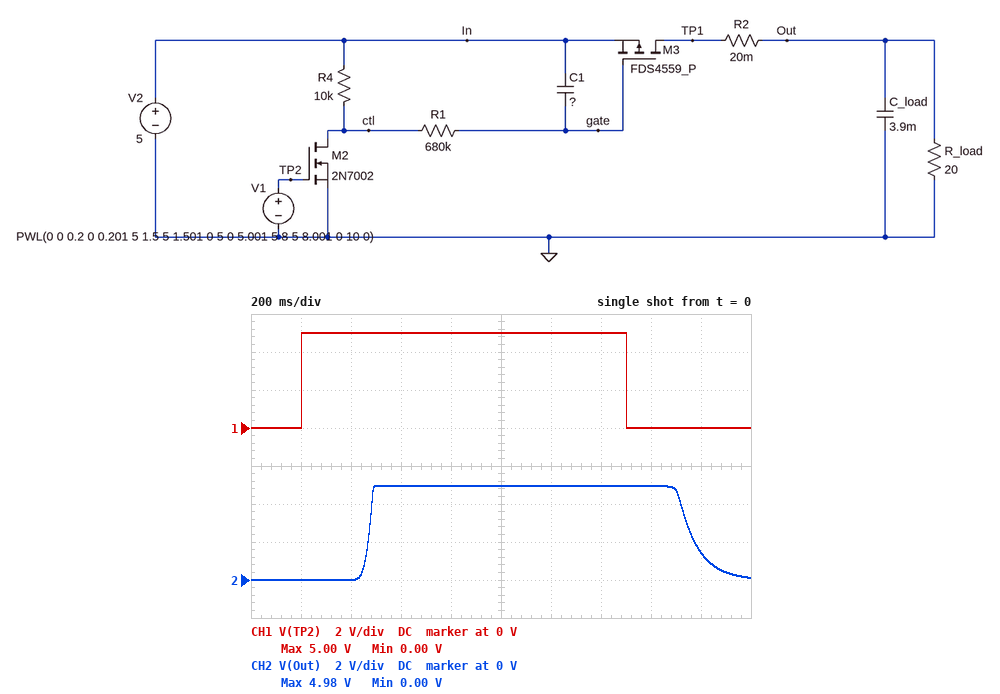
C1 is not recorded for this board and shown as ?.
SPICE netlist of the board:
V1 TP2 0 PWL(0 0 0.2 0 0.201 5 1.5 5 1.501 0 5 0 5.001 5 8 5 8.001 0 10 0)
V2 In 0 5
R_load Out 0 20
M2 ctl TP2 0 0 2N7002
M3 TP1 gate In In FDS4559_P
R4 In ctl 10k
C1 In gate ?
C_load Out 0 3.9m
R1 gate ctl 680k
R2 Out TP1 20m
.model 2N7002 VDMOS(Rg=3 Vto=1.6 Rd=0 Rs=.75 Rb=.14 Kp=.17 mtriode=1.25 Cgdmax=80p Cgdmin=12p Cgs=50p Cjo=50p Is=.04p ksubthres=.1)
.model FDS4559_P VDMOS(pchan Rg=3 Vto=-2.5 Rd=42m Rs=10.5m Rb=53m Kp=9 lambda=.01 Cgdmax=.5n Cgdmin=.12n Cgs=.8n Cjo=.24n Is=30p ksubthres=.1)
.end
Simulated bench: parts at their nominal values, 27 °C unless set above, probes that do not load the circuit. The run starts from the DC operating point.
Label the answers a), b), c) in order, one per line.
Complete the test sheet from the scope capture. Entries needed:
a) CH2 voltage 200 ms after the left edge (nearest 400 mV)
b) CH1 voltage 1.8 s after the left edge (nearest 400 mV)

a) 0 V
b) 0 V
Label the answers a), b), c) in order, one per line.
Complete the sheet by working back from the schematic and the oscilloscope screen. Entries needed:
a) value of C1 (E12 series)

a) 470 nF
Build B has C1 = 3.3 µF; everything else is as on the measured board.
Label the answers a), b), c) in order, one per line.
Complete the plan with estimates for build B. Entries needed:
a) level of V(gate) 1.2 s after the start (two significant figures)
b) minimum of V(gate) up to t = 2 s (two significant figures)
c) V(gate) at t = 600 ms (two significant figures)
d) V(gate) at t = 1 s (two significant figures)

a) 3.2 V
b) 2.8 V
c) 4.2 V
d) 3.5 V
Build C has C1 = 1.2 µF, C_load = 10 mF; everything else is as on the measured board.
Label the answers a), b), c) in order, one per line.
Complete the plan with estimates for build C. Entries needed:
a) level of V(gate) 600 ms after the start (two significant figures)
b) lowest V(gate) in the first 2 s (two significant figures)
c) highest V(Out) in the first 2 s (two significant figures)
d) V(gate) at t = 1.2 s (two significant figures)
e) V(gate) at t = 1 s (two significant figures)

a) 3.1 V
b) 1.0 V
c) 5.0 V
d) 1.5 V
e) 1.9 V
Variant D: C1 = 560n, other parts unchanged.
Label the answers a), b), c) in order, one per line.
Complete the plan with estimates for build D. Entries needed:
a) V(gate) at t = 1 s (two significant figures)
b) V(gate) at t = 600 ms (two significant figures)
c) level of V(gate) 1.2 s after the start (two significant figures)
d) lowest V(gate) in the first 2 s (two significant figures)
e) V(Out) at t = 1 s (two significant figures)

a) 620 mV
b) 1.8 V
c) 370 mV
d) 170 mV
e) 5.0 V
